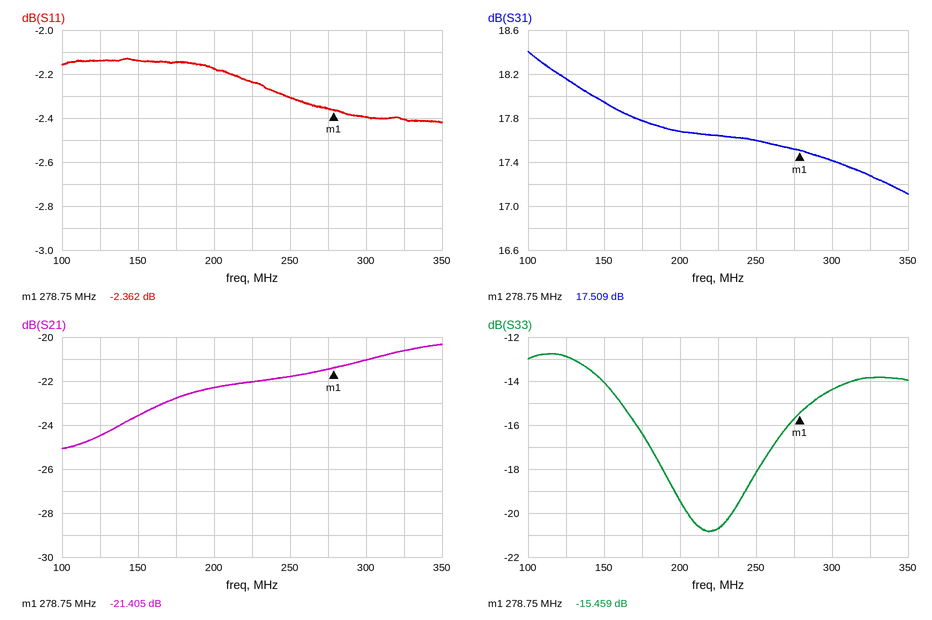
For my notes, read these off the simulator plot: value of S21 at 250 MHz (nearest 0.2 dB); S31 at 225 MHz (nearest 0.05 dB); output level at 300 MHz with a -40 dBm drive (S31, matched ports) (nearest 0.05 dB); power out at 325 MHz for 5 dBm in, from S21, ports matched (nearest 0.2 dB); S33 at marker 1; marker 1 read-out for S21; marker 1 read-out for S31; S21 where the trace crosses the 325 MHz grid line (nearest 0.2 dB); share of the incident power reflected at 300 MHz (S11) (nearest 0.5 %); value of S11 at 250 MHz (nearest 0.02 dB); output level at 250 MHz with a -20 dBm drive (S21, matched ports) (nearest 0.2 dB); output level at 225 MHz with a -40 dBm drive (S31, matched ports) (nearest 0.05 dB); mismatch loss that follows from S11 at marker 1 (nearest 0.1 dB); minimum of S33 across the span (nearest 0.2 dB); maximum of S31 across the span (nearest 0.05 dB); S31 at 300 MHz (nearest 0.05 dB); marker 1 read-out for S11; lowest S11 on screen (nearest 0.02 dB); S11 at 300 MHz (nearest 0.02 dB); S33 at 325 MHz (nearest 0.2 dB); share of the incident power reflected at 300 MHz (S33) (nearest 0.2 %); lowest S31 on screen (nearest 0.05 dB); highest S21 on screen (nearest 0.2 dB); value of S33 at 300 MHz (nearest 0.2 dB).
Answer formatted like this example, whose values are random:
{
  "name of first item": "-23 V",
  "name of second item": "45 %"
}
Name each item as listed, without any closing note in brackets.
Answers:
{
  "value of S21 at 250 MHz": "-21.8 dB",
  "S31 at 225 MHz": "17.65 dB",
  "output level at 300 MHz with a -40 dBm drive (S31, matched ports)": "-22.60 dBm",
  "power out at 325 MHz for 5 dBm in, from S21, ports matched": "-15.6 dBm",
  "S33 at marker 1": "-15.459 dB",
  "marker 1 read-out for S21": "-21.405 dB",
  "marker 1 read-out for S31": "17.509 dB",
  "S21 where the trace crosses the 325 MHz grid line": "-20.6 dB",
  "share of the incident power reflected at 300 MHz (S11)": "57.5 %",
  "value of S11 at 250 MHz": "-2.30 dB",
  "output level at 250 MHz with a -20 dBm drive (S21, matched ports)": "-41.8 dBm",
  "output level at 225 MHz with a -40 dBm drive (S31, matched ports)": "-22.35 dBm",
  "mismatch loss that follows from S11 at marker 1": "3.8 dB",
  "minimum of S33 across the span": "-20.8 dB",
  "maximum of S31 across the span": "18.40 dB",
  "S31 at 300 MHz": "17.40 dB",
  "marker 1 read-out for S11": "-2.362 dB",
  "lowest S11 on screen": "-2.42 dB",
  "S11 at 300 MHz": "-2.40 dB",
  "S33 at 325 MHz": "-13.8 dB",
  "share of the incident power reflected at 300 MHz (S33)": "3.6 %",
  "lowest S31 on screen": "17.10 dB",
  "highest S21 on screen": "-20.4 dB",
  "value of S33 at 300 MHz": "-14.4 dB"
}
